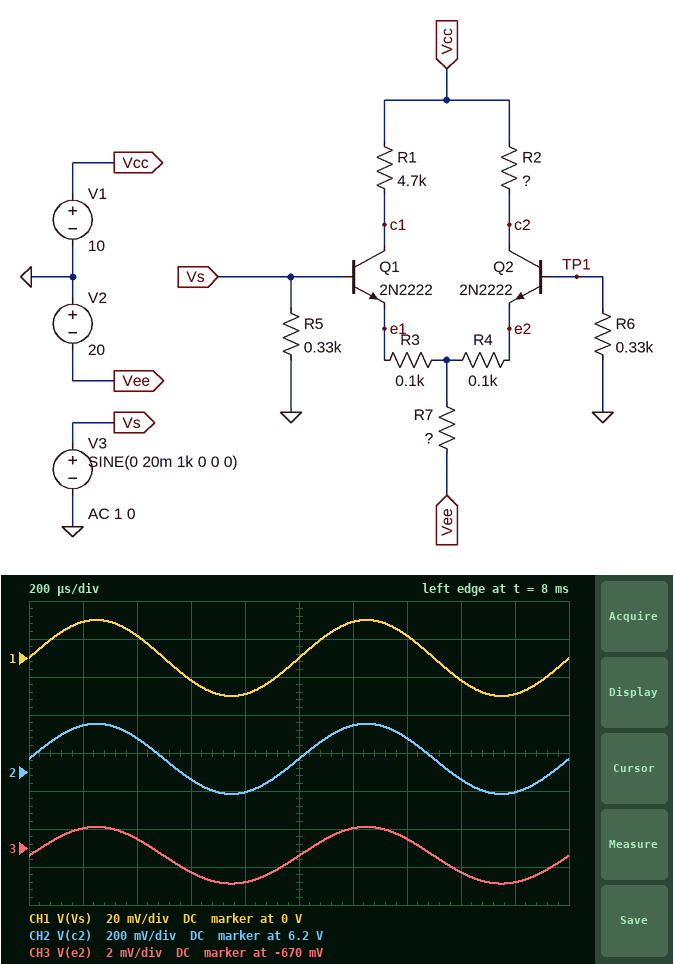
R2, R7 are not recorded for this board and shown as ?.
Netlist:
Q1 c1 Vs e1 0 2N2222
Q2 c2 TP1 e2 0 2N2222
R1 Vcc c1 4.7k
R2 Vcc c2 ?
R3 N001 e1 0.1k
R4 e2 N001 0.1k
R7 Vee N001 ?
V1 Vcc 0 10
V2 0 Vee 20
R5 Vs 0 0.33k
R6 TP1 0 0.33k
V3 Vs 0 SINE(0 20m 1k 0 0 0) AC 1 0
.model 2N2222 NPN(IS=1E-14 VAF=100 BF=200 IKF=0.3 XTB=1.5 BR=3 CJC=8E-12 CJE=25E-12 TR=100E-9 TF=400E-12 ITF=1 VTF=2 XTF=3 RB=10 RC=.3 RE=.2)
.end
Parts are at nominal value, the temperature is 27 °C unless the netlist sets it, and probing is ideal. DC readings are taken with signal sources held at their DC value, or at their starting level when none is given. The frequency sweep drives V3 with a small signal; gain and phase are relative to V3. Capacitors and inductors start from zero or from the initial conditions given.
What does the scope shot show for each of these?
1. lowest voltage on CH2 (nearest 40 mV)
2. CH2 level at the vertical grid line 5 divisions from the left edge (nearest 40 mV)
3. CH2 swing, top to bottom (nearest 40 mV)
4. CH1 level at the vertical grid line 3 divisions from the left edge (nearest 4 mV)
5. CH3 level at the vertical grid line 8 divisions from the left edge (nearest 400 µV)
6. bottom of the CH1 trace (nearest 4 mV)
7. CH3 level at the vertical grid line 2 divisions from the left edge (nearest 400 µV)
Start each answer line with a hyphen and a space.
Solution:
- 6.08 V
- 6.28 V
- 360 mV
- -12 mV
- -671.2 mV
- -20 mV
- -669.6 mV
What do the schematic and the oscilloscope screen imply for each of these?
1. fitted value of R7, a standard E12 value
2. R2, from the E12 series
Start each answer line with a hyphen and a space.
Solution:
- 5.6 kΩ
- 2.2 kΩ
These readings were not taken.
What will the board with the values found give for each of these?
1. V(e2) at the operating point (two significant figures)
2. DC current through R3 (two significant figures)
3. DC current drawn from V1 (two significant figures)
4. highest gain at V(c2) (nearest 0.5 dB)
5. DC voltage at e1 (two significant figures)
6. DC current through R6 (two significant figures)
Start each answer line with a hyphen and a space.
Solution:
- -670 mV
- 1.7 mA
- 3.4 mA
- 19.5 dB
- -670 mV
- 8.0 µA
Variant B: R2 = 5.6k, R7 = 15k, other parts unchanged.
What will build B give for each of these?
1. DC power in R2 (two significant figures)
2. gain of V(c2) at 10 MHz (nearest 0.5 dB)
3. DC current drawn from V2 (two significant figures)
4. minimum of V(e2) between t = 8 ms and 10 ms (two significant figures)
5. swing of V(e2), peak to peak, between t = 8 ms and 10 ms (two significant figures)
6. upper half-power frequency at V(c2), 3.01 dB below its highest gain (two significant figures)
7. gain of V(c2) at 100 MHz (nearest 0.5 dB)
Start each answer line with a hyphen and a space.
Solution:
- 2.3 mW
- 15.0 dB
- 1.3 mA
- -650 mV
- 6.1 mV
- 3.1 MHz
- -9.0 dB
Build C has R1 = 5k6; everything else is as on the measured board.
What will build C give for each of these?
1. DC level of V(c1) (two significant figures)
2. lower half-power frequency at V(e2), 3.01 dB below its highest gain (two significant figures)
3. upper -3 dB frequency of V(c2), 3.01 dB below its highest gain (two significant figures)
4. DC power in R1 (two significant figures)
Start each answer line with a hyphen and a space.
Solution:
- 440 mV
- 6.7 MHz
- 6.4 MHz
- 16 mW
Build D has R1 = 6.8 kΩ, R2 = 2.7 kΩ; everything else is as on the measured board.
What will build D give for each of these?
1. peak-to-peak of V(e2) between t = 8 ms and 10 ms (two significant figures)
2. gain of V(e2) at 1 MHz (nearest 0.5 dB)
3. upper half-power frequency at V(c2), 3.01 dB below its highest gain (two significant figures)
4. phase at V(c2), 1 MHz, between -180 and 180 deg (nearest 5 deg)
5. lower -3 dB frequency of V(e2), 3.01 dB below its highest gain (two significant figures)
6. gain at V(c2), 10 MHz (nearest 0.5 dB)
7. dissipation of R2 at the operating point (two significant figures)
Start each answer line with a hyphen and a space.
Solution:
- 2.5 mV
- -18.0 dB
- 6.0 MHz
- -5 deg
- 5.3 MHz
- 14.5 dB
- 8.0 mW
